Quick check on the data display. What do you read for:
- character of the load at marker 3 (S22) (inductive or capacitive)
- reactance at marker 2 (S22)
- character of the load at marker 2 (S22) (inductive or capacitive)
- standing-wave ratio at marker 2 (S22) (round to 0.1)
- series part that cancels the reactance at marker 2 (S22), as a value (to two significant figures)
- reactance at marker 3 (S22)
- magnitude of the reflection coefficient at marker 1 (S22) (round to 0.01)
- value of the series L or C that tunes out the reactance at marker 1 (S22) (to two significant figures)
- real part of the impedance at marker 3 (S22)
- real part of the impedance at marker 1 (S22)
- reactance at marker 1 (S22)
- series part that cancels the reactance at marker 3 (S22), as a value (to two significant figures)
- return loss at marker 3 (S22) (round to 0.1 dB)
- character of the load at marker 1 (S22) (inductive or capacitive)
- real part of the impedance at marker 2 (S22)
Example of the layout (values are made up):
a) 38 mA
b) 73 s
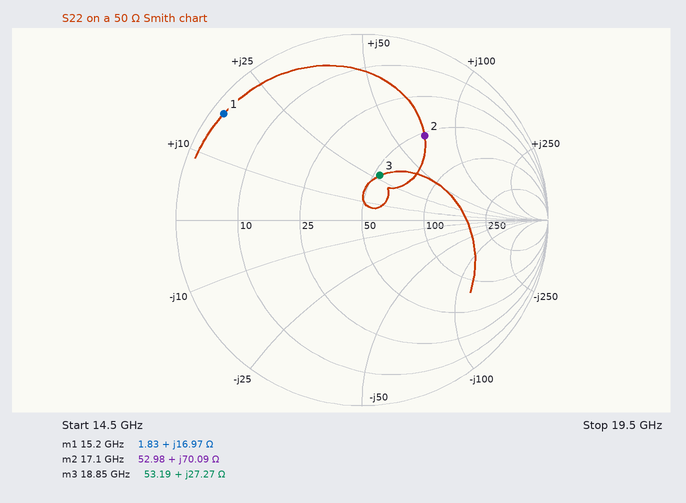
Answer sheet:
a) inductive
b) +70.09 Ω
c) inductive
d) 3.6
e) 130 fF
f) +27.27 Ω
g) 0.94
h) 620 fF
i) 53.19 Ω
j) 1.83 Ω
k) +16.97 Ω
l) 310 fF
m) 11.8 dB
n) inductive
o) 52.98 Ω
